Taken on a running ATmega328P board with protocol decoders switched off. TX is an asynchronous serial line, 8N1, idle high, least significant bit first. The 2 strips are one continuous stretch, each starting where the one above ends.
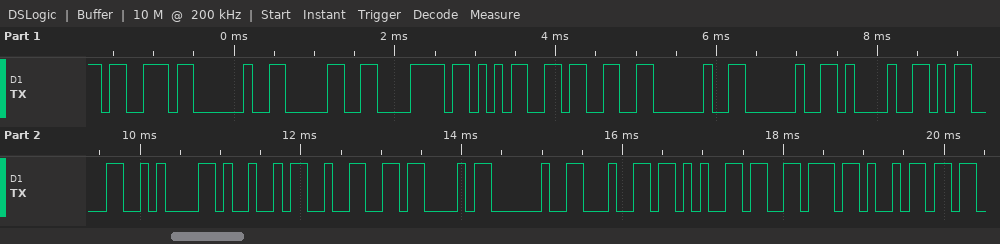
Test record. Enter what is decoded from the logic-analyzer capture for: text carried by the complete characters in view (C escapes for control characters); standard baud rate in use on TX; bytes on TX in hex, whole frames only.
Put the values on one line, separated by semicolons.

"s 0x53  !\r\nI2C devi"; 9600 baud; 73 20 30 78 35 33 20 20 21 0D 0A 49 32 43 20 64 65 76 69
